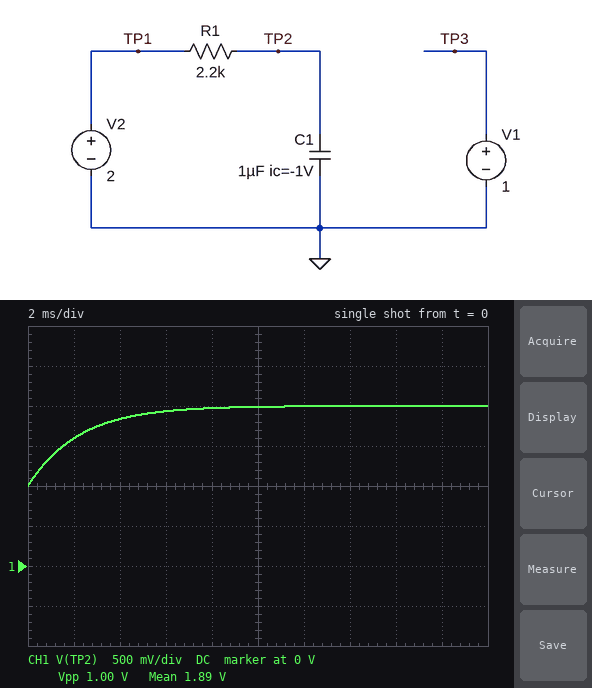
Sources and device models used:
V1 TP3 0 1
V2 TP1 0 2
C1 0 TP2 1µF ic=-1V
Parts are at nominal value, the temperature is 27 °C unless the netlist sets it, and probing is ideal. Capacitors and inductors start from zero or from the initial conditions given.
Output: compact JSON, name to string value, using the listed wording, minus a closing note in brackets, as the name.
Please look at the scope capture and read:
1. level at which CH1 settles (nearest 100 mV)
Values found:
{"level at which CH1 settles": "2.0 V"}
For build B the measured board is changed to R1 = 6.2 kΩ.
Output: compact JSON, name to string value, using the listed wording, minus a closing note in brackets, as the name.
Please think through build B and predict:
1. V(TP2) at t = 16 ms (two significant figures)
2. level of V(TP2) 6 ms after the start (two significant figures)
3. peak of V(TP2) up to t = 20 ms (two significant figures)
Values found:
{"V(TP2) at t = 16 ms": "1.9 V", "level of V(TP2) 6 ms after the start": "1.6 V", "peak of V(TP2) up to t = 20 ms": "2.0 V"}
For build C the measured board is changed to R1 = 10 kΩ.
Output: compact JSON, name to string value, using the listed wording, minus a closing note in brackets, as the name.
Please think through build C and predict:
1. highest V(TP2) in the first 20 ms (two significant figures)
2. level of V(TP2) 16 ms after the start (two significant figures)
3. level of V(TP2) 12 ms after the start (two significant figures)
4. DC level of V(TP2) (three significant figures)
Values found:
{"highest V(TP2) in the first 20 ms": "1.9 V", "level of V(TP2) 16 ms after the start": "1.8 V", "level of V(TP2) 12 ms after the start": "1.7 V", "DC level of V(TP2)": "2.00 V"}
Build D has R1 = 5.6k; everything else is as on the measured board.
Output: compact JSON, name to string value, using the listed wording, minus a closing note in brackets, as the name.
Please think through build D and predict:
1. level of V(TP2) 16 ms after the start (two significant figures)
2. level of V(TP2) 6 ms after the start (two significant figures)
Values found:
{"level of V(TP2) 16 ms after the start": "1.9 V", "level of V(TP2) 6 ms after the start": "1.7 V"}
